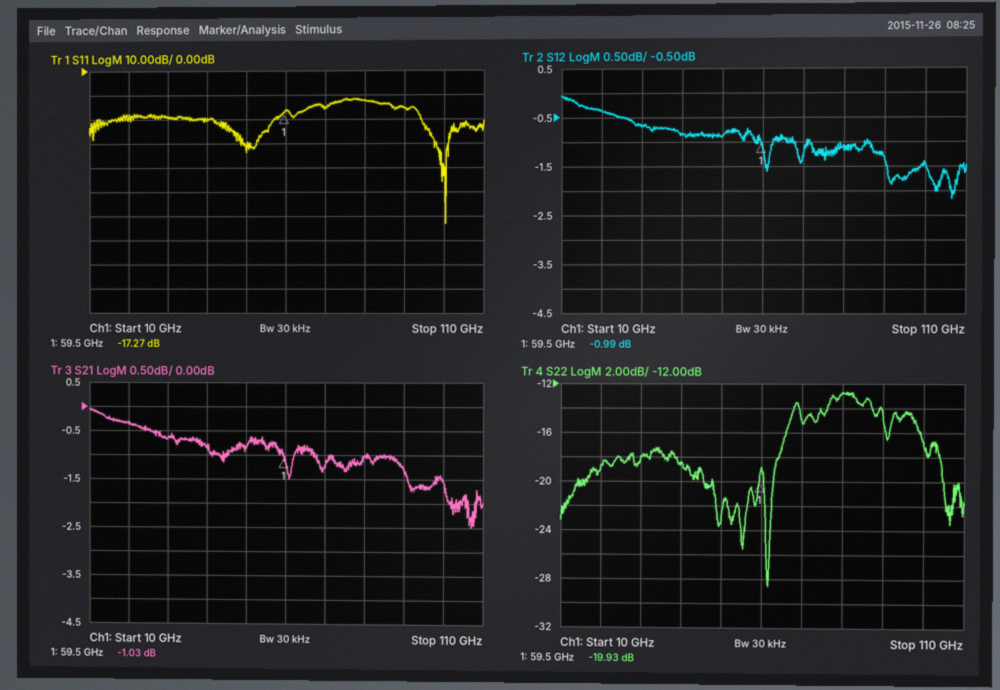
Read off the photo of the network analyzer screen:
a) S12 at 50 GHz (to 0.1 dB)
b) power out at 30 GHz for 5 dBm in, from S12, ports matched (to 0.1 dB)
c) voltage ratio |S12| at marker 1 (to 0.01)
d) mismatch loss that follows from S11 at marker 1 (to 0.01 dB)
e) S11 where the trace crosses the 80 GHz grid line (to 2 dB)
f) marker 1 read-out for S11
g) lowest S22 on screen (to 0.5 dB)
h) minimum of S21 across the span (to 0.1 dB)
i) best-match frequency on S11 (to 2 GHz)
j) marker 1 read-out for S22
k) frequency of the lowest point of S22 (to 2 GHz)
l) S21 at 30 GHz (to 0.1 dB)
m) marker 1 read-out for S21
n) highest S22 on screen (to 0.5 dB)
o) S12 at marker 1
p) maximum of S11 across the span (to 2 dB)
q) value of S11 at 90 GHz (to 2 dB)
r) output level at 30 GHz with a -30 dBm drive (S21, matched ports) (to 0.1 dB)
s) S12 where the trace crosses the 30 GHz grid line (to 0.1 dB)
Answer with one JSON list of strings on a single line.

["-0.9 dB", "4.3 dBm", "0.89", "0.08 dB", "-12 dB", "-17.27 dB", "-28.5 dB", "-2.5 dB", "100 GHz", "-19.93 dB", "62 GHz", "-0.7 dB", "-1.03 dB", "-12.5 dB", "-0.99 dB", "-12 dB", "-16 dB", "-30.7 dBm", "-0.7 dB"]
